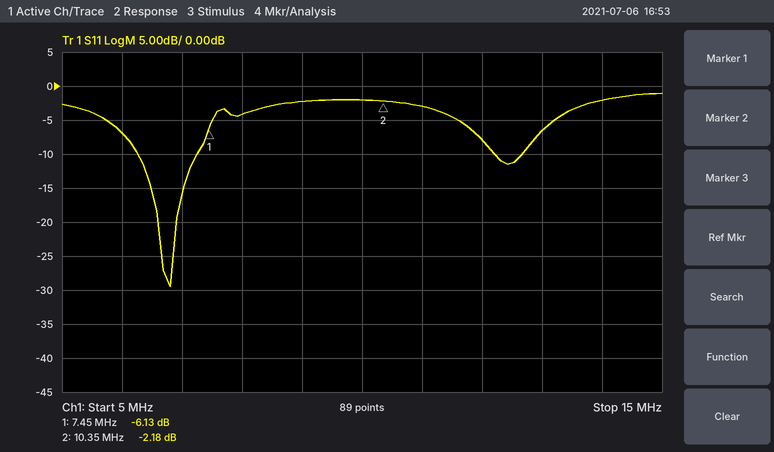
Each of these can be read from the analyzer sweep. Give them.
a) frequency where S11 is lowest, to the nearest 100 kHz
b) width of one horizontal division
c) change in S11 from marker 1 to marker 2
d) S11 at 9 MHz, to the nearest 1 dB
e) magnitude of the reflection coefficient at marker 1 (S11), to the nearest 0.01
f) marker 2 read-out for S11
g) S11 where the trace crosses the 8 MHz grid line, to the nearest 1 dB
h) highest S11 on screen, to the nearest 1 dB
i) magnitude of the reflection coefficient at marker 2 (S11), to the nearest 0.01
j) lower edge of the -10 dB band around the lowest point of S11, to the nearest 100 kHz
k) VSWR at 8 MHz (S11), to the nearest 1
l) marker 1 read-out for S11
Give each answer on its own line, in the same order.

6.8 MHz
1 MHz
3.95 dB
-2 dB
0.49
-2.18 dB
-4 dB
-1 dB
0.78
6.3 MHz
4
-6.13 dB
